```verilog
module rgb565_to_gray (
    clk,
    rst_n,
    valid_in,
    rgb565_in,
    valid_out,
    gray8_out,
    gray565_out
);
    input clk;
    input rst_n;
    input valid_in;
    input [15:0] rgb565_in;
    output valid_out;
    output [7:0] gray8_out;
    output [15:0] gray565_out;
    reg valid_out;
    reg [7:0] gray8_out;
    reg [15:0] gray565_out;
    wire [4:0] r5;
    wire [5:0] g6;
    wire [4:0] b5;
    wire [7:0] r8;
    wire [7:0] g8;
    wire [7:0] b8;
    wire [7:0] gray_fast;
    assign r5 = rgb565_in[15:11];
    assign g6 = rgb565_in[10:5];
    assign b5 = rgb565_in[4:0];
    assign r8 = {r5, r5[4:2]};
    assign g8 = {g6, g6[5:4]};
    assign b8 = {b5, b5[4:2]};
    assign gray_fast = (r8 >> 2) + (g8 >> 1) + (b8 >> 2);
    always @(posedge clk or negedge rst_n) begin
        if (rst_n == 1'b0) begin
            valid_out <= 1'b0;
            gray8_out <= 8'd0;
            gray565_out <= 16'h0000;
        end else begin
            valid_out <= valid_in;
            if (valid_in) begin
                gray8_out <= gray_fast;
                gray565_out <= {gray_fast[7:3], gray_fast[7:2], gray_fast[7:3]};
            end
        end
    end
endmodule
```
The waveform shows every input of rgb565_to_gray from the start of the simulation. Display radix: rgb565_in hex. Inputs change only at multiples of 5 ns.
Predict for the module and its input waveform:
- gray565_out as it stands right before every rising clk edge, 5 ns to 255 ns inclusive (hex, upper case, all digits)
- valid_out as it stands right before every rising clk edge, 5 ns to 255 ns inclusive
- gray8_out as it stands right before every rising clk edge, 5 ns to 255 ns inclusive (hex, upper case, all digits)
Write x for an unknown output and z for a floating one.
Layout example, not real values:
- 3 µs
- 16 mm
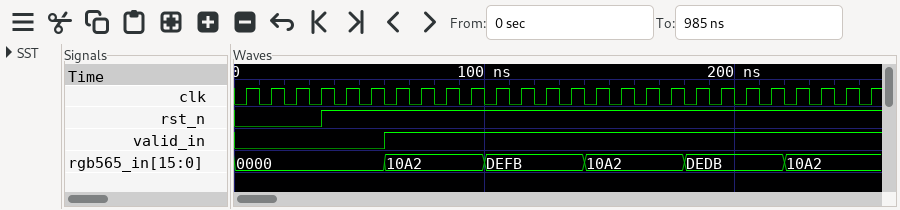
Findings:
- 0000, 0000, 0000, 0000, 0000, 0000, 0000, 1082, 1082, 1082, 1082, DEFB, DEFB, DEFB, DEFB, 1082, 1082, 1082, 1082, DEDB, DEDB, DEDB, DEDB, 1082, 1082, 1082
- 0 0 0 0 0 0 0 1 1 1 1 1 1 1 1 1 1 1 1 1 1 1 1 1 1 1
- 00, 00, 00, 00, 00, 00, 00, 12, 12, 12, 12, DD, DD, DD, DD, 12, 12, 12, 12, DB, DB, DB, DB, 12, 12, 12
